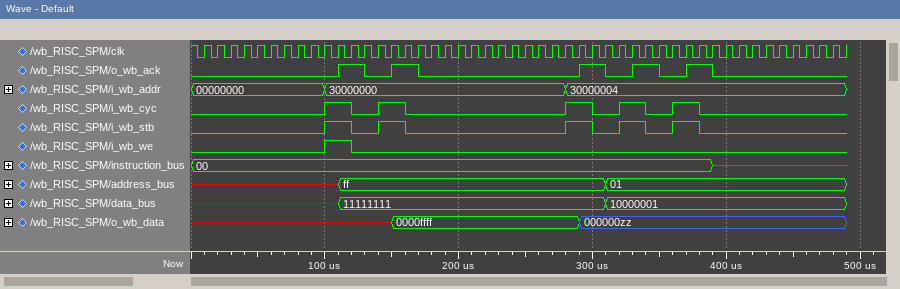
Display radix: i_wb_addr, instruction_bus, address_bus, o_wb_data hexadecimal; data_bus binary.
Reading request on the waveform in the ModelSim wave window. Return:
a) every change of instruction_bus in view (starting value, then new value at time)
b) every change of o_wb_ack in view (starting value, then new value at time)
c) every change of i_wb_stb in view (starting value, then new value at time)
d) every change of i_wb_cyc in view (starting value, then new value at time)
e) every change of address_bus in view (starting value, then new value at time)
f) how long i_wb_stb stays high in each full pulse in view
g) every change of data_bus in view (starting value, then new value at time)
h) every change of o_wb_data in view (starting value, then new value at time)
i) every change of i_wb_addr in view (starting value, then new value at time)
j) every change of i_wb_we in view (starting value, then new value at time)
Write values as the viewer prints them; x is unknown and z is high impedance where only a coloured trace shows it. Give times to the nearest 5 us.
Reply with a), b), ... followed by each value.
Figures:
a) 00, z at 390 us
b) 0, 1 at 110 us, 0 at 130 us, 1 at 150 us, 0 at 170 us, 1 at 290 us, 0 at 310 us, 1 at 330 us, 0 at 350 us, 1 at 370 us, 0 at 390 us
c) 0, 1 at 100 us, 0 at 120 us, 1 at 140 us, 0 at 160 us, 1 at 280 us, 0 at 300 us, 1 at 320 us, 0 at 340 us, 1 at 360 us, 0 at 380 us
d) 0, 1 at 100 us, 0 at 120 us, 1 at 140 us, 0 at 160 us, 1 at 280 us, 0 at 300 us, 1 at 320 us, 0 at 340 us, 1 at 360 us, 0 at 380 us
e) x, ff at 110 us, 01 at 310 us
f) 20 us, 20 us, 20 us, 20 us, 20 us
g) x, 11111111 at 110 us, 10000001 at 310 us
h) x, 0000ffff at 150 us, 000000zz at 290 us
i) 00000000, 30000000 at 100 us, 30000004 at 280 us
j) 0, 1 at 100 us, 0 at 120 us
